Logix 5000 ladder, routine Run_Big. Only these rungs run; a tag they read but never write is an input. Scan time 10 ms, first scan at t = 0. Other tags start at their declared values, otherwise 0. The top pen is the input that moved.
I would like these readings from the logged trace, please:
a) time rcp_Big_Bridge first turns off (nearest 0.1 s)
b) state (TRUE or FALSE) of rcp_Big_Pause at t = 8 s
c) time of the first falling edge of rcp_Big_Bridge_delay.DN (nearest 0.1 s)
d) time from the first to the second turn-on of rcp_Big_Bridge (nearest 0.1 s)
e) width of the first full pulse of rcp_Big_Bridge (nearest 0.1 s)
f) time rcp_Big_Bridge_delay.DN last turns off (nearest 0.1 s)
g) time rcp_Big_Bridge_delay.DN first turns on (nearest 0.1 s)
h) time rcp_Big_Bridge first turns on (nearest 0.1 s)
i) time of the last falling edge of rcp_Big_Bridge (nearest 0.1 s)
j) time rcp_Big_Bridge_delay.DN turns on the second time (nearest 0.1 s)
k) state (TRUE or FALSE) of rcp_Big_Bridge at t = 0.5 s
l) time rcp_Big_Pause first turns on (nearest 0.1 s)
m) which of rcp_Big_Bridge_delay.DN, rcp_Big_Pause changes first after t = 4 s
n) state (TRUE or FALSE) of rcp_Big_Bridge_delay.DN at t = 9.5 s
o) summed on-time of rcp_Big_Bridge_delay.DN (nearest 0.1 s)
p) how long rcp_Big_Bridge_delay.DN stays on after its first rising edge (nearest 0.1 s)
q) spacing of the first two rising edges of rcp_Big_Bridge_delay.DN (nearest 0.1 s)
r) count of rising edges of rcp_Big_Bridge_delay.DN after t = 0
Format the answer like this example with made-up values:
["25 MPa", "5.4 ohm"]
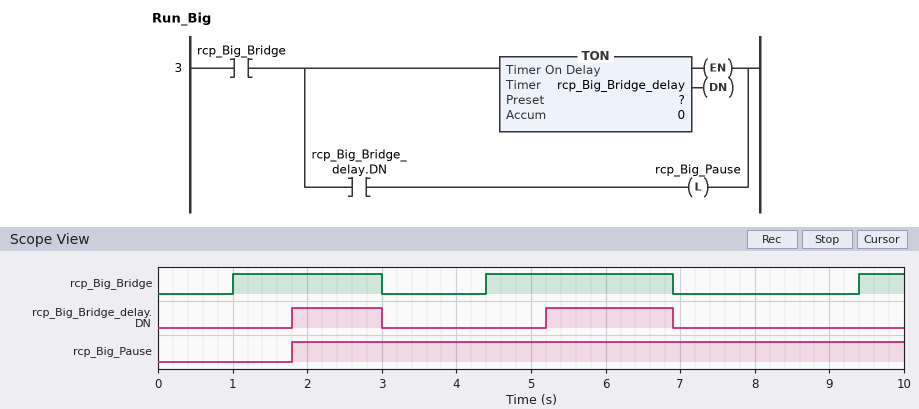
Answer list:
["3.0 s", "TRUE", "3.0 s", "3.4 s", "2.0 s", "6.9 s", "1.8 s", "1.0 s", "6.9 s", "5.2 s", "FALSE", "1.8 s", "rcp_Big_Bridge_delay.DN", "FALSE", "2.9 s", "1.2 s", "3.4 s", "2"]
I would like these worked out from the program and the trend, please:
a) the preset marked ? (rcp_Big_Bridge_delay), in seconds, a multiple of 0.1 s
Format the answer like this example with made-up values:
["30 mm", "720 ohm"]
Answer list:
["0.8 s"]
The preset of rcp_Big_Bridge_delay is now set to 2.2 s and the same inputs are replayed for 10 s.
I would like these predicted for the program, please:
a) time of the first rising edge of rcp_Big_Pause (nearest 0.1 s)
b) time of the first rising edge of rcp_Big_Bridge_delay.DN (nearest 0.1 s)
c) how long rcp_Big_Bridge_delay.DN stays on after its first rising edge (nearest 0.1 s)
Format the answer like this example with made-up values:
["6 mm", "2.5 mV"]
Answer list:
["6.6 s", "6.6 s", "0.3 s"]
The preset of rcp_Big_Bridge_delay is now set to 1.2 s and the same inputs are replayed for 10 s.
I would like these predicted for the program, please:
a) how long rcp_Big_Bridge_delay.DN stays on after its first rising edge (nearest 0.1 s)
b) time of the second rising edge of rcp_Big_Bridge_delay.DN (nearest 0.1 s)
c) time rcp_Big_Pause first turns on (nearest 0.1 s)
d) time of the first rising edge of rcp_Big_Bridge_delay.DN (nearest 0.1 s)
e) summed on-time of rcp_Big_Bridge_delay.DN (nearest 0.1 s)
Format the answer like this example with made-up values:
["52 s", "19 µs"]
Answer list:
["0.8 s", "5.6 s", "2.2 s", "2.2 s", "2.1 s"]
